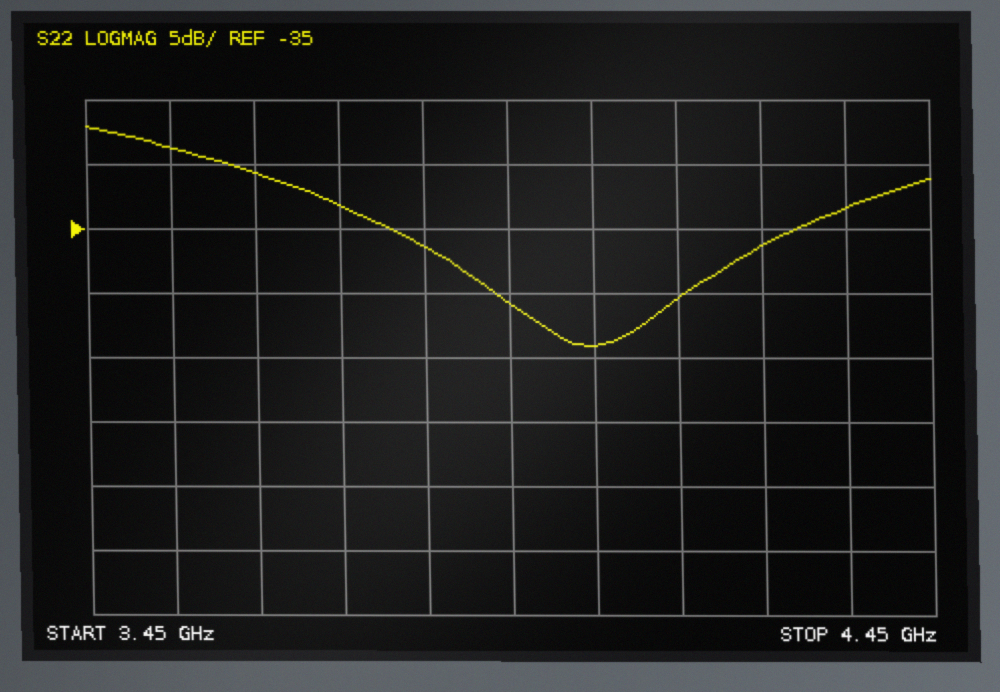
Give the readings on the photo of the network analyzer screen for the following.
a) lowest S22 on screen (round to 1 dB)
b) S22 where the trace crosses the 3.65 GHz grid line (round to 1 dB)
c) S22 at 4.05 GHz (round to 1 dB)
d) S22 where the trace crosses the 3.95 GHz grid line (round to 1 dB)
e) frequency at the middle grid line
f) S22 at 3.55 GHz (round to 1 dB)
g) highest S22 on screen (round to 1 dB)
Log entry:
-44 dB
-31 dB
-44 dB
-41 dB
3.95 GHz
-29 dB
-27 dB
